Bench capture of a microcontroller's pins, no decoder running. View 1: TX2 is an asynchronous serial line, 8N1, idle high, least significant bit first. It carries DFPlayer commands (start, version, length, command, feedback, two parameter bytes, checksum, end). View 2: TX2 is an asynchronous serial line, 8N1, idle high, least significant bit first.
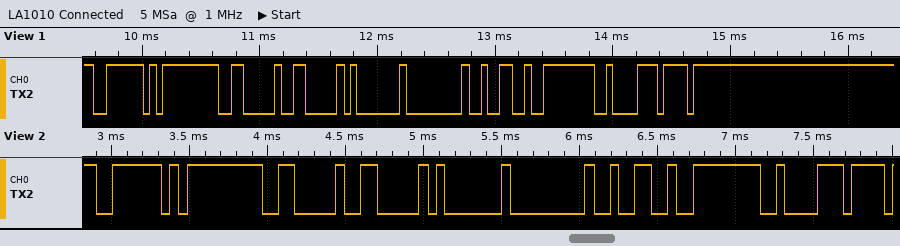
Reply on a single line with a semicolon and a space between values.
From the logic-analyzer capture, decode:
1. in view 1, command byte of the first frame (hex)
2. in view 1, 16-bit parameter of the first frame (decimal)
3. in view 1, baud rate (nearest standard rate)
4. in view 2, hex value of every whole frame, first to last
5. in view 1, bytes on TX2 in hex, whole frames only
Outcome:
0x06; 50; 19200 baud; 7E FF 06 06 01 00 32 FE C2; 7E FF 06 06 01 00 32 FE C2 EF
